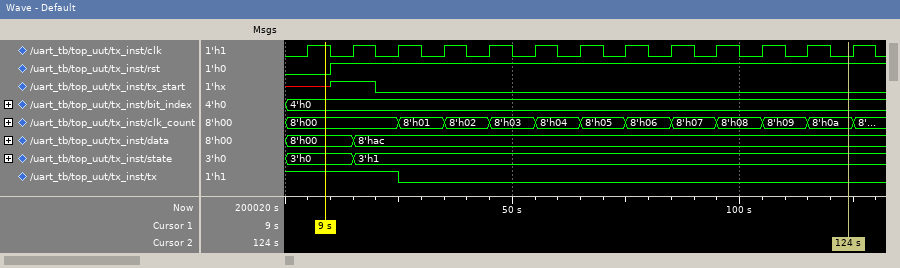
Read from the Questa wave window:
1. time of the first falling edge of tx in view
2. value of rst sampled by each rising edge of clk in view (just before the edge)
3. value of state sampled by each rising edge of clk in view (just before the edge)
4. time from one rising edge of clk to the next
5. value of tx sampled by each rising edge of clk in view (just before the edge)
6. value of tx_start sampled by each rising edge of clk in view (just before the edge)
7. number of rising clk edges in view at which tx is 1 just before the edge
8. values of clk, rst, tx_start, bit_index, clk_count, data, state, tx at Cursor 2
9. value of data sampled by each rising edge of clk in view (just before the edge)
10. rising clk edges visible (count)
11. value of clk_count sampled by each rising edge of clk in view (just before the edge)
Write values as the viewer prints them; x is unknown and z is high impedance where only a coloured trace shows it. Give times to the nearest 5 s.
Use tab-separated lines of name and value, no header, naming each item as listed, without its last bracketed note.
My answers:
time of the first falling edge of tx in view	25 s
value of rst sampled by each rising edge of clk in view	0 1 1 1 1 1 1 1 1 1 1 1 1
value of state sampled by each rising edge of clk in view	3'h0, 3'h0, 3'h1, 3'h1, 3'h1, 3'h1, 3'h1, 3'h1, 3'h1, 3'h1, 3'h1, 3'h1, 3'h1
time from one rising edge of clk to the next	10 s
value of tx sampled by each rising edge of clk in view	1 1 1 0 0 0 0 0 0 0 0 0 0
value of tx_start sampled by each rising edge of clk in view	x 1 0 0 0 0 0 0 0 0 0 0 0
number of rising clk edges in view at which tx is 1 just before the edge	3
values of clk, rst, tx_start, bit_index, clk_count, data, state, tx at Cursor 2	clk=0, rst=1, tx_start=0, bit_index=4'h0, clk_count=8'h0a, data=8'hac, state=3'h1, tx=0
value of data sampled by each rising edge of clk in view	8'h00, 8'h00, 8'hac, 8'hac, 8'hac, 8'hac, 8'hac, 8'hac, 8'hac, 8'hac, 8'hac, 8'hac, 8'hac
rising clk edges visible	13
value of clk_count sampled by each rising edge of clk in view	8'h00, 8'h00, 8'h00, 8'h01, 8'h02, 8'h03, 8'h04, 8'h05, 8'h06, 8'h07, 8'h08, 8'h09, 8'h0a
